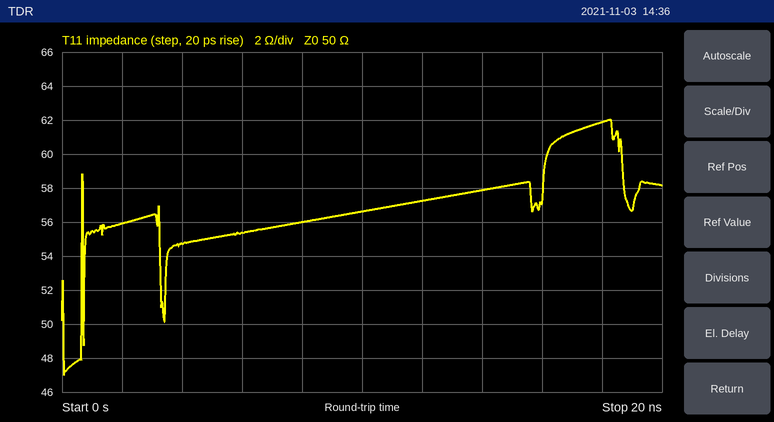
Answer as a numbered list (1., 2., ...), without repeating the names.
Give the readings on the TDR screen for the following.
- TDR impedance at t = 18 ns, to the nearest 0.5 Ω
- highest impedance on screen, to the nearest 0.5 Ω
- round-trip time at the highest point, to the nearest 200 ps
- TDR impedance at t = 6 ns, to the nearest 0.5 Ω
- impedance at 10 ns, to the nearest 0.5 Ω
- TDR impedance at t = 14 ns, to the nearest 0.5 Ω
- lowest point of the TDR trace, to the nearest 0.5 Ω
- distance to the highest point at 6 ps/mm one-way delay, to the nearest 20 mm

1. 62.0 Ω
2. 62.0 Ω
3. 18.2 ns
4. 55.5 Ω
5. 56.5 Ω
6. 58.0 Ω
7. 47.0 Ω
8. 1.52 m
